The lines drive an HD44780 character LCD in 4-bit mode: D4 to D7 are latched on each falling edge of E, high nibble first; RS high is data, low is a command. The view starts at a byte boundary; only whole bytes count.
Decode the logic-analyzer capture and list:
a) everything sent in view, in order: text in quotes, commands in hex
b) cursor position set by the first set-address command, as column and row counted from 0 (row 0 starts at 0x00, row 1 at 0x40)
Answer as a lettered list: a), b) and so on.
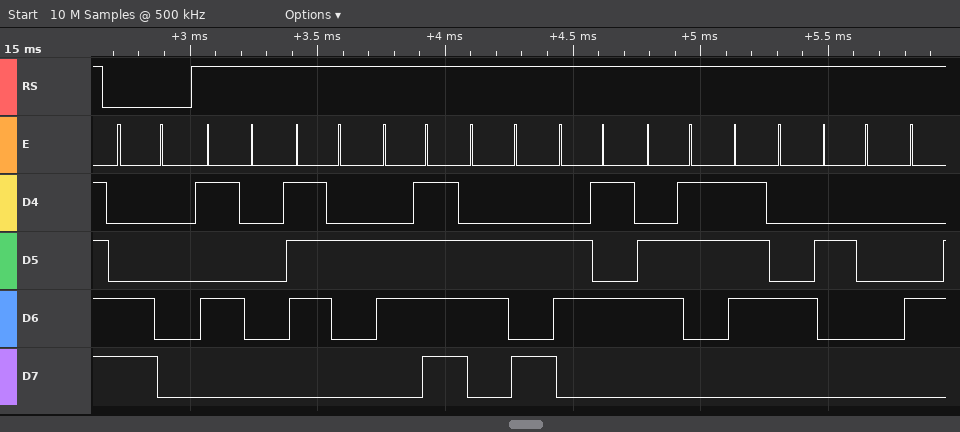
a) 0xC0 "Project "
b) column 0, row 1
